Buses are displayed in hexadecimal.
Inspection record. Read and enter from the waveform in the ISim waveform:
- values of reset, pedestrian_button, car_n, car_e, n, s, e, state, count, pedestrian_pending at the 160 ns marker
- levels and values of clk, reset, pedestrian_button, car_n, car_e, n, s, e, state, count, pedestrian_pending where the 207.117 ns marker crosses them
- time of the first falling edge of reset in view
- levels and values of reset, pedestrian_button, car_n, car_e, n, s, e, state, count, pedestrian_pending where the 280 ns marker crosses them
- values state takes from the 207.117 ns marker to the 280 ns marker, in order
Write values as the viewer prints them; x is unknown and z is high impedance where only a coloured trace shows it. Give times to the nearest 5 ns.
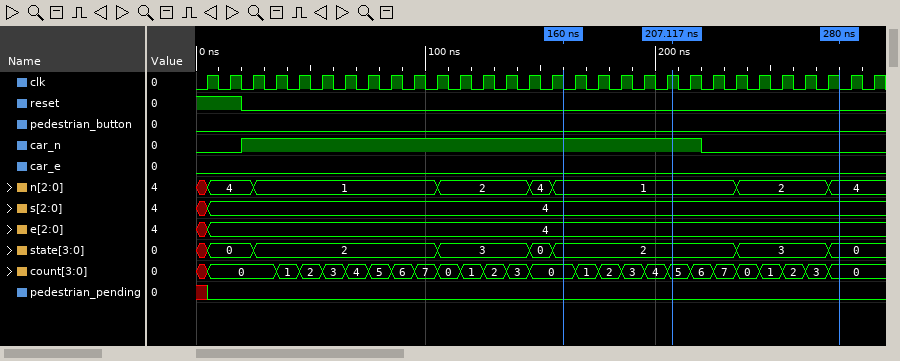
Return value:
reset=0, pedestrian_button=0, car_n=1, car_e=0, n=1, s=4, e=4, state=2, count=0, pedestrian_pending=0
clk=1, reset=0, pedestrian_button=0, car_n=1, car_e=0, n=1, s=4, e=4, state=2, count=5, pedestrian_pending=0
20 ns
reset=0, pedestrian_button=0, car_n=0, car_e=0, n=4, s=4, e=4, state=0, count=0, pedestrian_pending=0
2, 3, 0
